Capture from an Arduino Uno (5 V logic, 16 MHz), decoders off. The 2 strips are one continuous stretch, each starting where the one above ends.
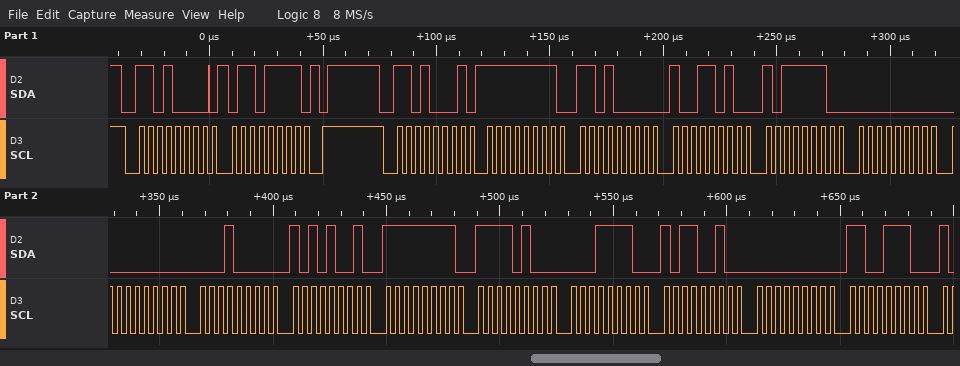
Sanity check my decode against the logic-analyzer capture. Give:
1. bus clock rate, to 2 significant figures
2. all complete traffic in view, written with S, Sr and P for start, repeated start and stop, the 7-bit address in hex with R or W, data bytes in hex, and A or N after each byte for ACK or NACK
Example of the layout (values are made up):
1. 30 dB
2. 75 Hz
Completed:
1. 250 kHz
2. S 68W A 6F A P S 68R A FF A D0 A 9A A BE A 00 A 00 A 10 A A9 A FF A F4 A 1E A B2 A 00 A CE A
